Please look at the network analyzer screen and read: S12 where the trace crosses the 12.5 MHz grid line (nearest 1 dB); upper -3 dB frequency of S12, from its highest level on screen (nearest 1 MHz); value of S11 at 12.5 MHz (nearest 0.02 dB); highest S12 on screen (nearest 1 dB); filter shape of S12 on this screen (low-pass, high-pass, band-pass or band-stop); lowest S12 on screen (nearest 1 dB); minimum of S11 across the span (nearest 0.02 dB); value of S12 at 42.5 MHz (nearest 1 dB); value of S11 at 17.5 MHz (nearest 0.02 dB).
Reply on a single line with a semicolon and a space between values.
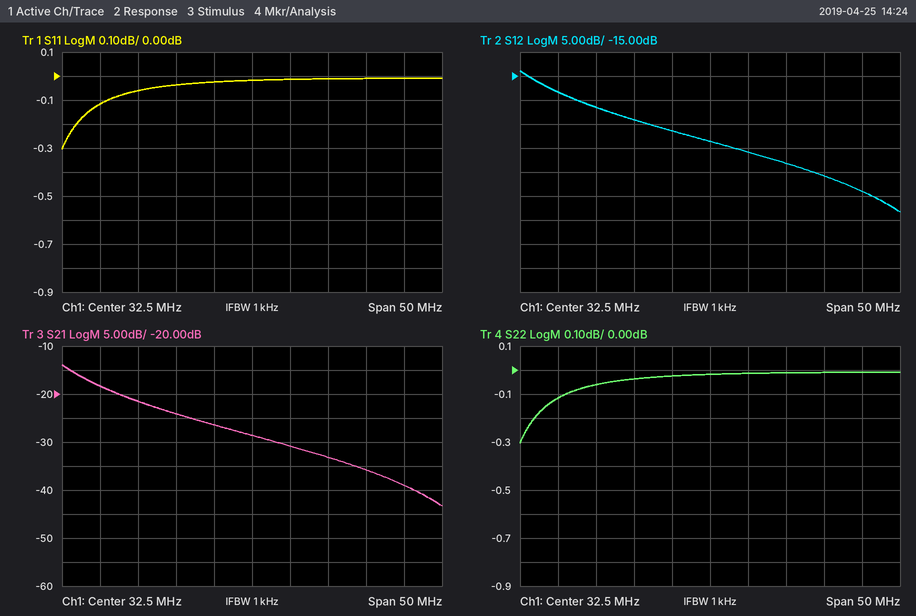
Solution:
-18 dB; 11 MHz; -0.12 dB; -14 dB; low-pass; -43 dB; -0.30 dB; -33 dB; -0.06 dB
